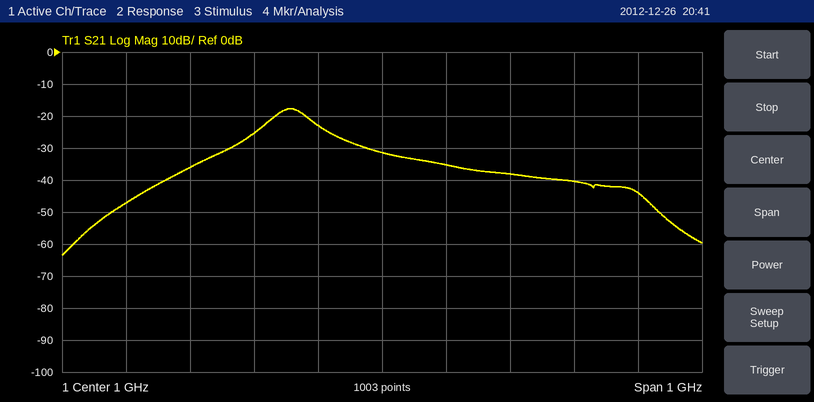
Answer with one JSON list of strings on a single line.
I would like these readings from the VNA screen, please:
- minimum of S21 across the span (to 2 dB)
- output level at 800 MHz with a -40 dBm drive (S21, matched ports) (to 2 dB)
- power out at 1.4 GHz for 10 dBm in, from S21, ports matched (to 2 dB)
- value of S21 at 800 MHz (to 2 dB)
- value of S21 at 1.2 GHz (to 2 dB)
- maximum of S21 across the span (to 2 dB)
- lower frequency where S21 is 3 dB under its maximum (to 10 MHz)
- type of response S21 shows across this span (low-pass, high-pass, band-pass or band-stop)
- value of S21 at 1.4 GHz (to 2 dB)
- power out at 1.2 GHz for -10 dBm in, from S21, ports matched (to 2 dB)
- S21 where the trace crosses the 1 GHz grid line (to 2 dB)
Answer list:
["-64 dB", "-66 dBm", "-34 dBm", "-26 dB", "-38 dB", "-18 dB", "830 MHz", "band-pass", "-44 dB", "-48 dBm", "-32 dB"]
